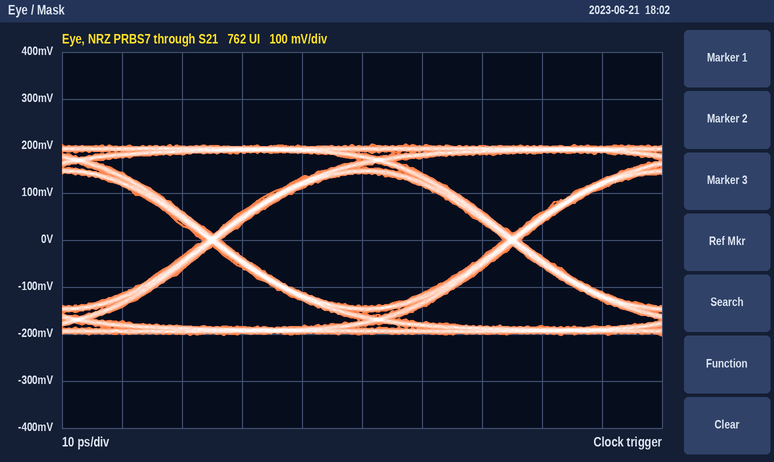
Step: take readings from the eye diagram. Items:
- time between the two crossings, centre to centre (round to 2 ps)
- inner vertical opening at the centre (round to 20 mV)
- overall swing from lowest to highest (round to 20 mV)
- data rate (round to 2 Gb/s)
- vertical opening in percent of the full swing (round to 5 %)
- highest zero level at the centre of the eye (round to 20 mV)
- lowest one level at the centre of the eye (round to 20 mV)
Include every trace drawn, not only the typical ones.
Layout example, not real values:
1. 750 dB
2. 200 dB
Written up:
1. 50 ps
2. 280 mV
3. 400 mV
4. 20 Gb/s
5. 70 %
6. -140 mV
7. 140 mV
